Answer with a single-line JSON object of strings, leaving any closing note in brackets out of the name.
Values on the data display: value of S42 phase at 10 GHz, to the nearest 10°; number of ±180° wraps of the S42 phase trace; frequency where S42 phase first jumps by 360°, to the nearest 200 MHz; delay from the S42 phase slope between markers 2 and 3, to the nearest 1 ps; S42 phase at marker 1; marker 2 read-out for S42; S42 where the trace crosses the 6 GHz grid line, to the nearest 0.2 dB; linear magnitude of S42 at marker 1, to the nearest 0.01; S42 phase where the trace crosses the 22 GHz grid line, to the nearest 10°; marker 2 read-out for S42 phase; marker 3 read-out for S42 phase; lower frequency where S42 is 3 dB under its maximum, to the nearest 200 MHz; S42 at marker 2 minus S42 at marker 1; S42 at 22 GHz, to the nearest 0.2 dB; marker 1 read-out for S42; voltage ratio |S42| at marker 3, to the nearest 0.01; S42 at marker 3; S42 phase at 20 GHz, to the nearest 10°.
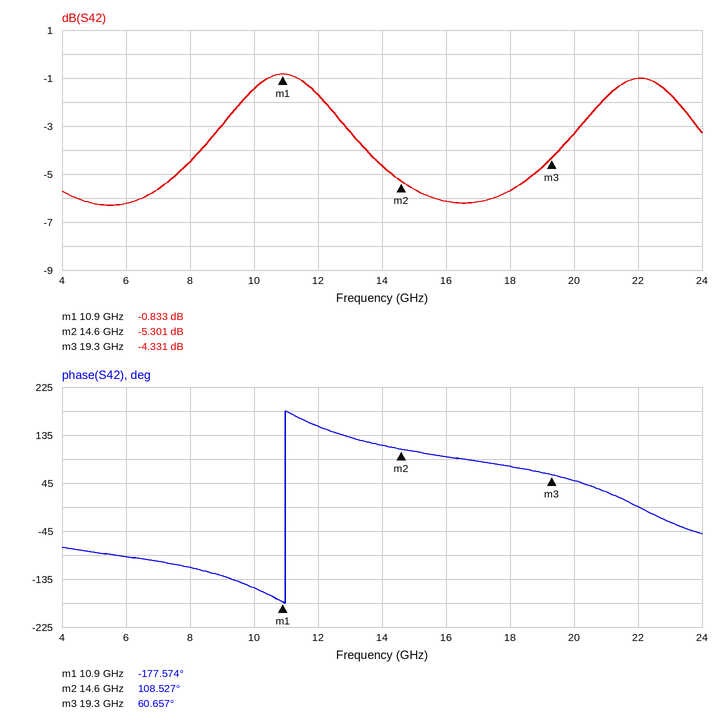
{"value of S42 phase at 10 GHz, to the nearest 10°": "-150°", "number of ±180° wraps of the S42 phase trace": "1", "frequency where S42 phase first jumps by 360°, to the nearest 200 MHz": "11.0 GHz", "delay from the S42 phase slope between markers 2 and 3, to the nearest 1 ps": "28 ps", "S42 phase at marker 1": "-177.574°", "marker 2 read-out for S42": "-5.301 dB", "S42 where the trace crosses the 6 GHz grid line, to the nearest 0.2 dB": "-6.2 dB", "linear magnitude of S42 at marker 1, to the nearest 0.01": "0.91", "S42 phase where the trace crosses the 22 GHz grid line, to the nearest 10°": "0°", "marker 2 read-out for S42 phase": "108.527°", "marker 3 read-out for S42 phase": "60.657°", "lower frequency where S42 is 3 dB under its maximum, to the nearest 200 MHz": "8.4 GHz", "S42 at marker 2 minus S42 at marker 1": "-4.468 dB", "S42 at 22 GHz, to the nearest 0.2 dB": "-1.0 dB", "marker 1 read-out for S42": "-0.833 dB", "voltage ratio |S42| at marker 3, to the nearest 0.01": "0.61", "S42 at marker 3": "-4.331 dB", "S42 phase at 20 GHz, to the nearest 10°": "50°"}
